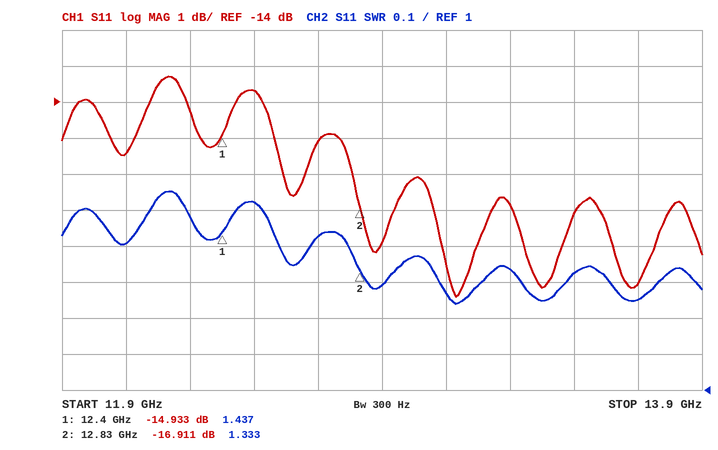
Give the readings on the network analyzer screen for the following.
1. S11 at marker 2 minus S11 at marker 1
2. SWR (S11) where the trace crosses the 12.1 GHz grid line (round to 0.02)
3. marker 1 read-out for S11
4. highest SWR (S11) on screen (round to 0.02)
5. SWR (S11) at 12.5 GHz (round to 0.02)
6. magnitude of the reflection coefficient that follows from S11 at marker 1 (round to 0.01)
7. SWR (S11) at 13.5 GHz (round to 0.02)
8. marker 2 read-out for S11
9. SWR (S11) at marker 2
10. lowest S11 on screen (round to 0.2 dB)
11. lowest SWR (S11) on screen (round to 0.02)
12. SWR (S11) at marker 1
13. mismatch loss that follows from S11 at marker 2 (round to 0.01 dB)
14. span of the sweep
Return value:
-1.978 dB
1.40
-14.933 dB
1.56
1.52
0.18
1.32
-16.911 dB
1.333
-19.4 dB
1.24
1.437
0.09 dB
2 GHz
